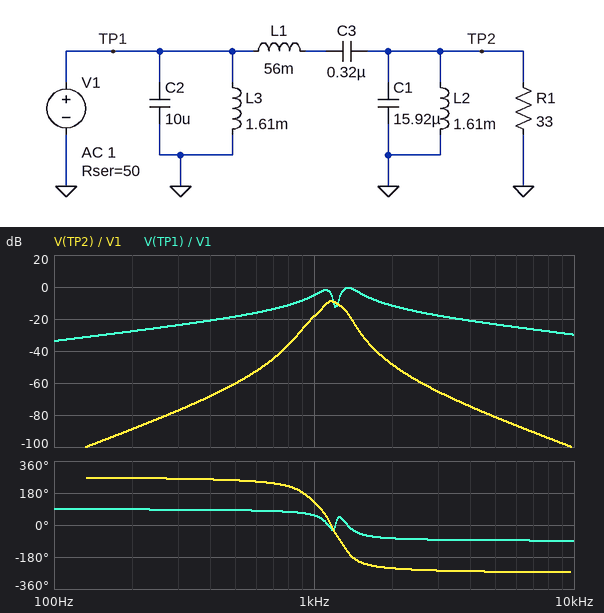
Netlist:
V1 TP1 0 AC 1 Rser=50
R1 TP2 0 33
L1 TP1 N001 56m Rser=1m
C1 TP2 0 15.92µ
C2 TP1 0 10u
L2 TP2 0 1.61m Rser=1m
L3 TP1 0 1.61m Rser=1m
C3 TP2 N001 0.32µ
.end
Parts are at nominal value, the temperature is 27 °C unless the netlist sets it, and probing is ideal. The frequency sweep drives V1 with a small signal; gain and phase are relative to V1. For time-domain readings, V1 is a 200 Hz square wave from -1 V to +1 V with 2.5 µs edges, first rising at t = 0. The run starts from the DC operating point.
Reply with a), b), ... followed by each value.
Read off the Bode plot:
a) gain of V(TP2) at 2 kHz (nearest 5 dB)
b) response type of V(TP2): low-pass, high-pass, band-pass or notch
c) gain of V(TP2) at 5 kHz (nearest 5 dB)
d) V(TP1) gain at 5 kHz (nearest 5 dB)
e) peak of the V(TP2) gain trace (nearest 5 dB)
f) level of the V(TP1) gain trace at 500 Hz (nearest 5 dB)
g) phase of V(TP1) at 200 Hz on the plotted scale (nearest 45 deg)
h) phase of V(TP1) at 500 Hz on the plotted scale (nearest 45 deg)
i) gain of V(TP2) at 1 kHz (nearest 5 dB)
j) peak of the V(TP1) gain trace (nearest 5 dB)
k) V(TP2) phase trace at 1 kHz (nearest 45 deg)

a) -50 dB
b) band-pass
c) -80 dB
d) -25 dB
e) -10 dB
f) -20 dB
g) 90 deg
h) 90 deg
i) -20 dB
j) 0 dB
k) 135 deg
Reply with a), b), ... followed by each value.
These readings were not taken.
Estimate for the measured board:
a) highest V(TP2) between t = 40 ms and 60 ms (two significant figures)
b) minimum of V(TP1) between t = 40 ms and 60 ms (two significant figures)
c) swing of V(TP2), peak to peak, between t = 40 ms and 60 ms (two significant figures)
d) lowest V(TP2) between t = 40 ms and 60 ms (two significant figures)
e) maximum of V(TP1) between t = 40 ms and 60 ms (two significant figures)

a) 46 mV
b) -460 mV
c) 92 mV
d) -46 mV
e) 460 mV
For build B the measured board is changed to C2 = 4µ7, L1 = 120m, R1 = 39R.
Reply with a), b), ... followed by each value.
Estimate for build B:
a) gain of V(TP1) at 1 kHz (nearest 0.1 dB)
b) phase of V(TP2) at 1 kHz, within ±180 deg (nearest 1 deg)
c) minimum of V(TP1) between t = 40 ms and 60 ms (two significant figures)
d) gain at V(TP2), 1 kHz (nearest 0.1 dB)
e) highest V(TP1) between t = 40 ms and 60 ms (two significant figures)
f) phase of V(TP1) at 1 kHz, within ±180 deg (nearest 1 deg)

a) -11.6 dB
b) -10 deg
c) -570 mV
d) -28.0 dB
e) 570 mV
f) 74 deg
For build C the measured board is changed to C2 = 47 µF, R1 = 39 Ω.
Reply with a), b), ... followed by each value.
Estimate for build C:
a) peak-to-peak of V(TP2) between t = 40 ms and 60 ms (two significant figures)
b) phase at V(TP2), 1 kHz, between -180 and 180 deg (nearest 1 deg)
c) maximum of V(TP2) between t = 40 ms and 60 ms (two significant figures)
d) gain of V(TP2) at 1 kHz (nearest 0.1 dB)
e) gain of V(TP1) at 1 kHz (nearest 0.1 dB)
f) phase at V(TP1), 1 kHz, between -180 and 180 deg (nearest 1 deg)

a) 23 mV
b) -11 deg
c) 12 mV
d) -32.0 dB
e) -20.2 dB
f) -84 deg
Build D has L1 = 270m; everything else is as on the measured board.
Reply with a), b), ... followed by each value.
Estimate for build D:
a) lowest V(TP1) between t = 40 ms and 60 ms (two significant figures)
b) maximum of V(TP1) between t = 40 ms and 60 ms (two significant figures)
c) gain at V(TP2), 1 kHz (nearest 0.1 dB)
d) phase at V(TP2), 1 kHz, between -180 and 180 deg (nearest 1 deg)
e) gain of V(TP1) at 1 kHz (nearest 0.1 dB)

a) -390 mV
b) 390 mV
c) -37.6 dB
d) -29 deg
e) -6.4 dB
